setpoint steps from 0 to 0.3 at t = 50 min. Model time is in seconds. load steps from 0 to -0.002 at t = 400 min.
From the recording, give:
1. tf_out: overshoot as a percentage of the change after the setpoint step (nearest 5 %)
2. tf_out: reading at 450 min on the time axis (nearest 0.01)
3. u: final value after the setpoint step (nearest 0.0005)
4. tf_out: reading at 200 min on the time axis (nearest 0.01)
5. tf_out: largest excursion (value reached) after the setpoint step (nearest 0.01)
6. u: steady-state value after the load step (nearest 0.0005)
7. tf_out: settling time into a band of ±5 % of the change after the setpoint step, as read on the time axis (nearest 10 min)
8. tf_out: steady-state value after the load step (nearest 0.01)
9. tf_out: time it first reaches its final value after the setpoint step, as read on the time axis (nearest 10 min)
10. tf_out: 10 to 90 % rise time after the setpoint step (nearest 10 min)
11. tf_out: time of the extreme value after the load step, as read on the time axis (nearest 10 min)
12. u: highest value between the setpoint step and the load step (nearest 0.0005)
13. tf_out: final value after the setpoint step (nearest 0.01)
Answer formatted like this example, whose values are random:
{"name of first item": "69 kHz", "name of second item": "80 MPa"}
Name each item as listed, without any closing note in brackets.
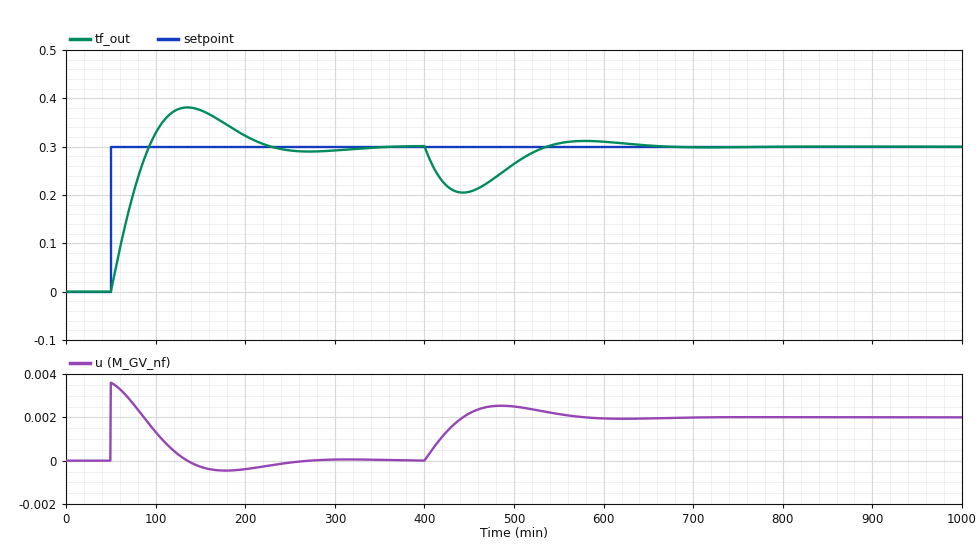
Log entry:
{"tf_out: overshoot as a percentage of the change after the setpoint step": "25 %", "tf_out: reading at 450 min on the time axis": "0.21", "u: final value after the setpoint step": "0.0000", "tf_out: reading at 200 min on the time axis": "0.32", "tf_out: largest excursion (value reached) after the setpoint step": "0.38", "u: steady-state value after the load step": "0.0020", "tf_out: settling time into a band of ±5 % of the change after the setpoint step, as read on the time axis": "210 min", "tf_out: steady-state value after the load step": "0.30", "tf_out: time it first reaches its final value after the setpoint step, as read on the time axis": "90 min", "tf_out: 10 to 90 % rise time after the setpoint step": "30 min", "tf_out: time of the extreme value after the load step, as read on the time axis": "440 min", "u: highest value between the setpoint step and the load step": "0.0035", "tf_out: final value after the setpoint step": "0.30"}
